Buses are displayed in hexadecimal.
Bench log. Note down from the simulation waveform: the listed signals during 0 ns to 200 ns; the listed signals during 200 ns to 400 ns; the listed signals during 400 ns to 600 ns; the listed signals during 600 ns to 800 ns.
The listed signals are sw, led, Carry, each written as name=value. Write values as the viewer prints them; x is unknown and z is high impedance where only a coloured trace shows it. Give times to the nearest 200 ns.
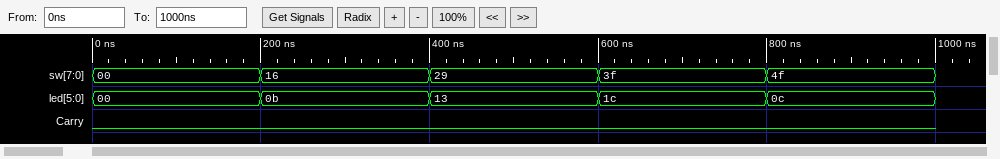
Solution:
sw=00, led=00, Carry=0
sw=16, led=0b, Carry=0
sw=29, led=13, Carry=0
sw=3f, led=1c, Carry=0
